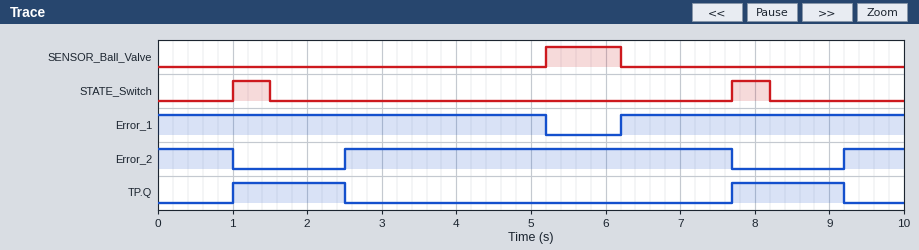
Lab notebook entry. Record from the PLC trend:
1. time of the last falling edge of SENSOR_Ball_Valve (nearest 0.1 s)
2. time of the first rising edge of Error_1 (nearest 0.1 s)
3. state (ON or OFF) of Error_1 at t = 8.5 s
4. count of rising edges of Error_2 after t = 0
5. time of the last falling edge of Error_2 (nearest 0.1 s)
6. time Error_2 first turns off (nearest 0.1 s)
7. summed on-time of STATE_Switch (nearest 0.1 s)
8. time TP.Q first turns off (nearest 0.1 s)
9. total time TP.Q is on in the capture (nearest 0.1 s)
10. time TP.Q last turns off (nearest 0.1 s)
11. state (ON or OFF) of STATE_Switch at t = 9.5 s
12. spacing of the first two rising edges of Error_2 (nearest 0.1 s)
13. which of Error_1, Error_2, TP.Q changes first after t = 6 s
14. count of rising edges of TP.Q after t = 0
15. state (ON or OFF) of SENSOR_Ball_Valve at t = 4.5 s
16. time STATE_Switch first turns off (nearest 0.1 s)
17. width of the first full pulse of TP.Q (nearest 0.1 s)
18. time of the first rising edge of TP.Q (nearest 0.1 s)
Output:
6.2 s
6.2 s
ON
2
7.7 s
1.0 s
1.0 s
2.5 s
3.0 s
9.2 s
OFF
6.7 s
Error_1
2
OFF
1.5 s
1.5 s
1.0 s
